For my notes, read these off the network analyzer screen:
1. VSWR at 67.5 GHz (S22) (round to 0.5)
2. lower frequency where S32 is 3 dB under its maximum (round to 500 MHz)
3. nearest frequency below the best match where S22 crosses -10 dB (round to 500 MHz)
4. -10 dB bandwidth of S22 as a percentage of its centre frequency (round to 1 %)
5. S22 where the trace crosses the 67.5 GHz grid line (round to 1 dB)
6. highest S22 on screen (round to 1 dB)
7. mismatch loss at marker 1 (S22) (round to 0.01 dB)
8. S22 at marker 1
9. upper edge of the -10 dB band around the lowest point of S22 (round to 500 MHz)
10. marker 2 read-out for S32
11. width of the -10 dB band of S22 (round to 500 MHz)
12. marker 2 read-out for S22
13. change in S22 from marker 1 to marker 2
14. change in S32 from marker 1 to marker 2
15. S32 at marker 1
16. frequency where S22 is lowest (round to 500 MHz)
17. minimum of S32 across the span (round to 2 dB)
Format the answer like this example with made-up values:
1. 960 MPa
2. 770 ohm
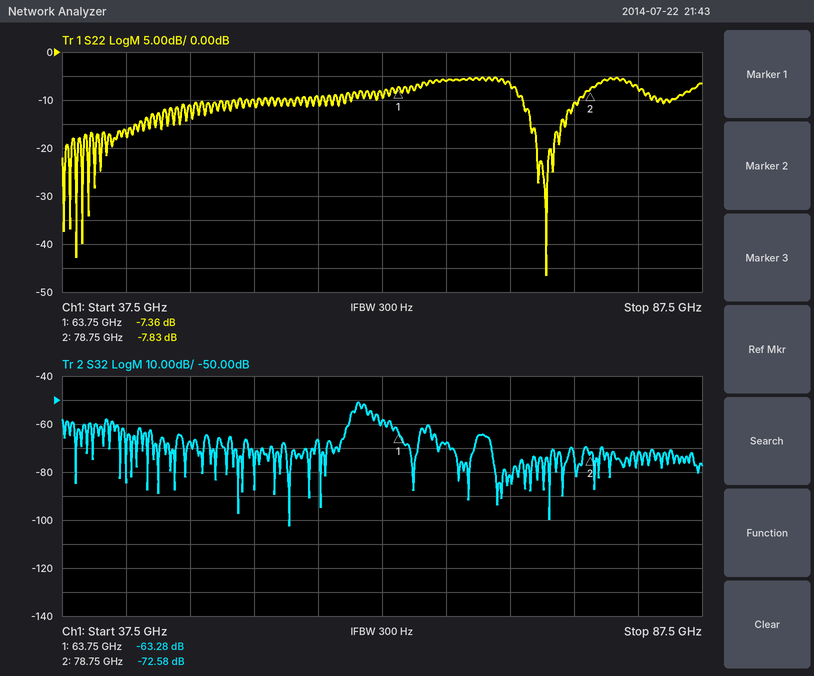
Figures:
1. 3.0
2. 60.5 GHz
3. 73.5 GHz
4. 6 %
5. -6 dB
6. -5 dB
7. 0.88 dB
8. -7.36 dB
9. 78.0 GHz
10. -72.58 dB
11. 4.5 GHz
12. -7.83 dB
13. -0.47 dB
14. -9.30 dB
15. -63.28 dB
16. 75.5 GHz
17. -102 dB
